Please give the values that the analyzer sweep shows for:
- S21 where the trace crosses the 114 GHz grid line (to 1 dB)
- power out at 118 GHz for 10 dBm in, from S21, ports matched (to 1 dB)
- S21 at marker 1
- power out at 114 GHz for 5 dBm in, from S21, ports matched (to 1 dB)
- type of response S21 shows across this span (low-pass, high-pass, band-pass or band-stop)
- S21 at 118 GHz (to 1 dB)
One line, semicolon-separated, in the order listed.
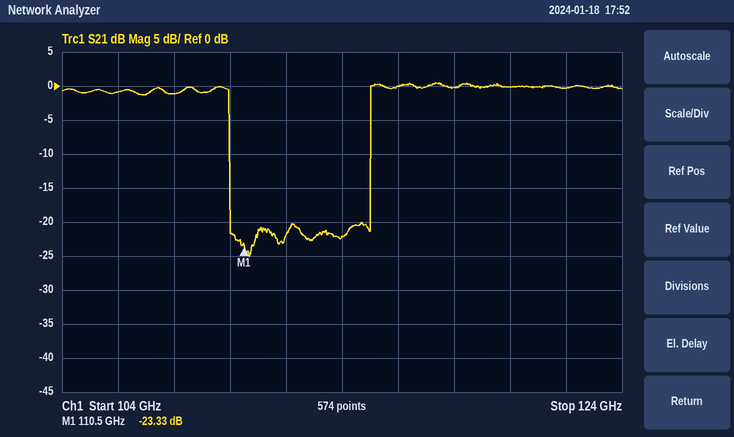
-22 dB; 10 dBm; -23.33 dB; -17 dBm; band-stop; 0 dB
